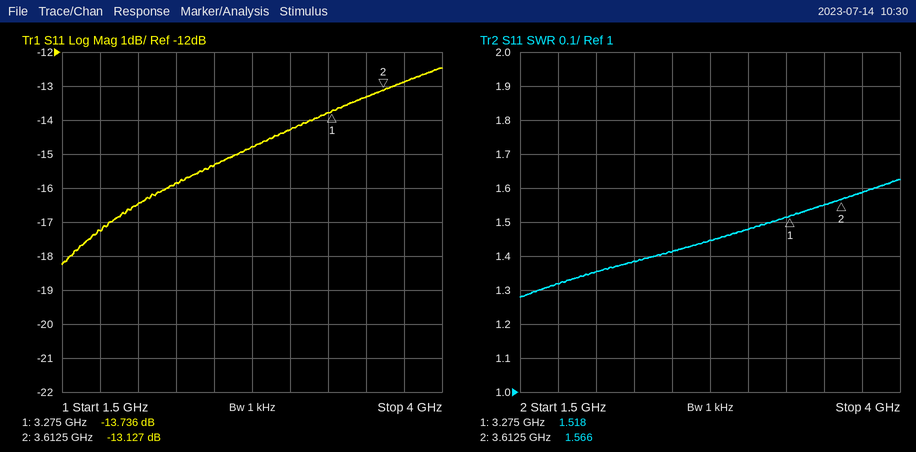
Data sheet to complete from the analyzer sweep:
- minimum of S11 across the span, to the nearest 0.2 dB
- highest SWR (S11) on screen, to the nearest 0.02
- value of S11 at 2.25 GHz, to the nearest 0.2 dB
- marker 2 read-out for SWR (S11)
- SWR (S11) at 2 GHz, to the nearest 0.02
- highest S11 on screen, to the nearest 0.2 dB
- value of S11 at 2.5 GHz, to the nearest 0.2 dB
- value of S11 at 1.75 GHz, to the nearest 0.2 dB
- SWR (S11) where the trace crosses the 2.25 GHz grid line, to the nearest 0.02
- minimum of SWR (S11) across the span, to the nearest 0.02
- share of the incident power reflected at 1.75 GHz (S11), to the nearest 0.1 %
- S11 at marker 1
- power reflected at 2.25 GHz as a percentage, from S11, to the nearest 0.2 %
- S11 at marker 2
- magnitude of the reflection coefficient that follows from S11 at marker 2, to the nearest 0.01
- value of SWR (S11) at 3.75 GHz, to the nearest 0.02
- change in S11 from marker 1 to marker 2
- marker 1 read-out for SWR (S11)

-18.2 dB
1.62
-15.8 dB
1.566
1.36
-12.4 dB
-15.4 dB
-17.2 dB
1.38
1.28
1.9 %
-13.736 dB
2.6 %
-13.127 dB
0.22
1.58
0.609 dB
1.518
